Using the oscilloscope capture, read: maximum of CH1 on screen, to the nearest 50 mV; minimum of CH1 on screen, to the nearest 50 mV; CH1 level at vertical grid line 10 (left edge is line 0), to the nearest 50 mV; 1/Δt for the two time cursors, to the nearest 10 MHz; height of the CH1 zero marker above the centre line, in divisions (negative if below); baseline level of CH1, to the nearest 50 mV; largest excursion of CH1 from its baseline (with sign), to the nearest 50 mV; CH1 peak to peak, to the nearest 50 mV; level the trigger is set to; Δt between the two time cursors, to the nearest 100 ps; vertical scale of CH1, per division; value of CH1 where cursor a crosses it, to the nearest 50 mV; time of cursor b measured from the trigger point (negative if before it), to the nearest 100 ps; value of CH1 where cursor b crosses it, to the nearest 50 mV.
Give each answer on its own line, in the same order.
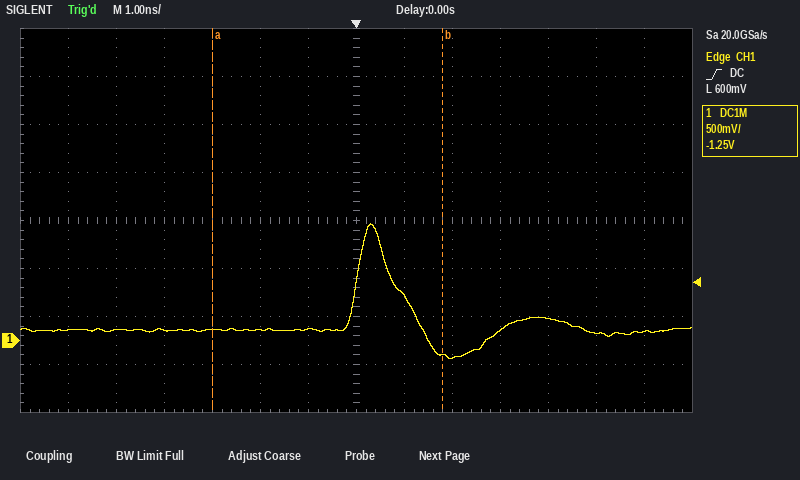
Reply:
1.20 V
-200 mV
100 mV
210 MHz
-2.5 div
100 mV
+1.10 V
1.40 V
600 mV
4.8 ns
500 mV
100 mV
+1.8 ns
-150 mV
